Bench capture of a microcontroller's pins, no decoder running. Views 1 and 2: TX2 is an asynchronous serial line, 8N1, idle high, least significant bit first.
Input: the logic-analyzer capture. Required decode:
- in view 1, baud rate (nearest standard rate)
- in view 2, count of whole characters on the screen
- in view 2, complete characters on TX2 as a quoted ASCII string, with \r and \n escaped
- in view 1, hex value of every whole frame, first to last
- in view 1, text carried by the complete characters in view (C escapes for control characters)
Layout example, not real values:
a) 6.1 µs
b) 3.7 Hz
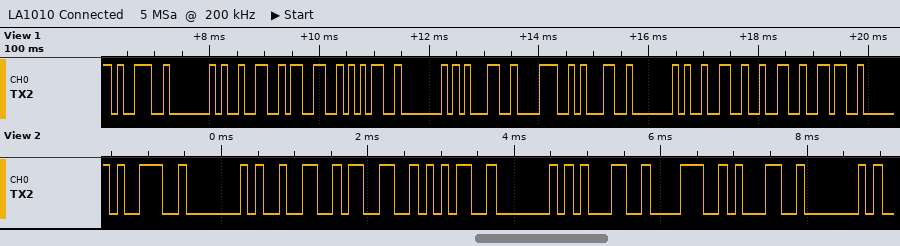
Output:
a) 9600 baud
b) 10
c) "9@235@181@"
d) 39 40 32 33 35 40 31 38 31 40 32 32 36
e) "9@235@181@226"
